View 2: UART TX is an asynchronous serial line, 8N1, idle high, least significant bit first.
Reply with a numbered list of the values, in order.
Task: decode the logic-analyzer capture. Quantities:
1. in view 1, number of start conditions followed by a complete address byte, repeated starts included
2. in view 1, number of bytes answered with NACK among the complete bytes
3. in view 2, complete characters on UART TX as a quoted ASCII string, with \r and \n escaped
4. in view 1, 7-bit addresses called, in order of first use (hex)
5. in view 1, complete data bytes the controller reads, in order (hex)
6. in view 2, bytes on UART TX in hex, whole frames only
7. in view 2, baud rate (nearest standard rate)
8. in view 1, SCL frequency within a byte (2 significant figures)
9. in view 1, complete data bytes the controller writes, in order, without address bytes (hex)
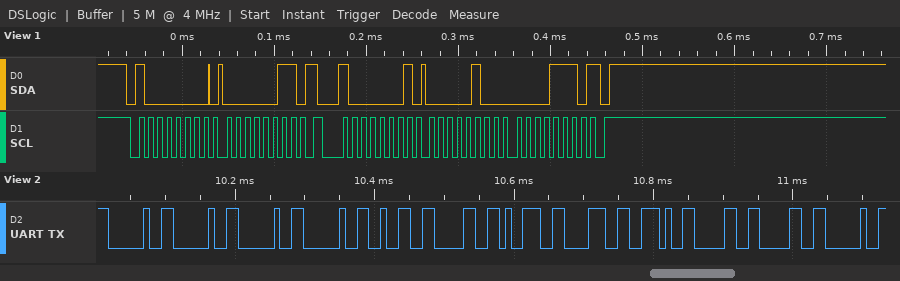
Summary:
1. 2
2. 1
3. "    2098.00 "
4. 0x40
5. 04 0E
6. 0x20 0x20 0x20 0x20 0x32 0x30 0x39 0x38 0x2E 0x30 0x30 0x20
7. 115200 baud
8. 100 kHz
9. 03
